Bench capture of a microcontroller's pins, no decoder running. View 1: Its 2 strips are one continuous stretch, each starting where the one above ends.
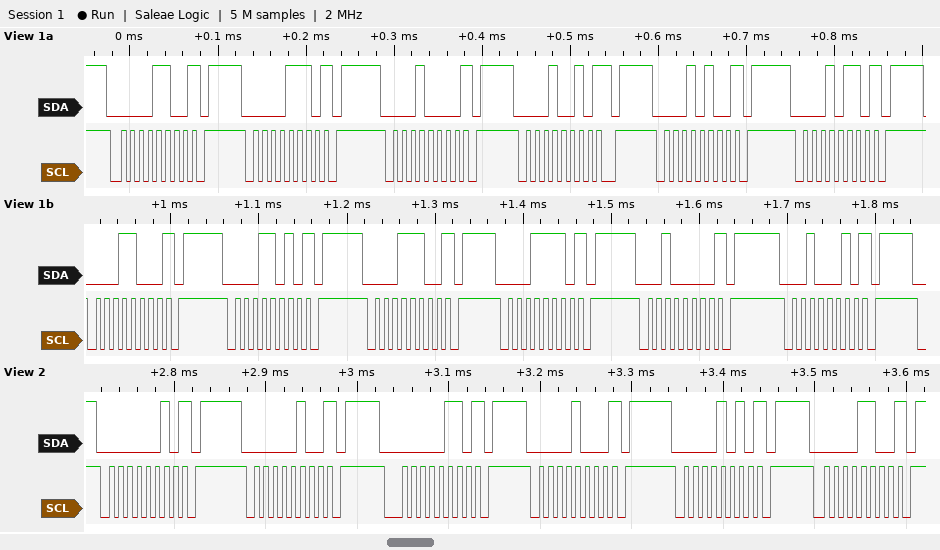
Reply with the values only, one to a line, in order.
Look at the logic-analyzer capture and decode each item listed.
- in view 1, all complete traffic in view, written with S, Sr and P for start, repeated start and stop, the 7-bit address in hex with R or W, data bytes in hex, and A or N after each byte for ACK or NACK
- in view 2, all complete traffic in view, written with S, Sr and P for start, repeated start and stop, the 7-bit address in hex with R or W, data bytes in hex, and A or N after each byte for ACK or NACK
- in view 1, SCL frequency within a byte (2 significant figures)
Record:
S 06W N P S 07W N P S 08W N P S 09W N P S 0AW N P S 0BW N P S 0CW N P S 0DW N P S 0EW N P S 0FW N P S 10W N P S 11W N P
S 01W N P S 02W N P S 03W N P S 04W N P S 05W N P S 06W N P
100 kHz
